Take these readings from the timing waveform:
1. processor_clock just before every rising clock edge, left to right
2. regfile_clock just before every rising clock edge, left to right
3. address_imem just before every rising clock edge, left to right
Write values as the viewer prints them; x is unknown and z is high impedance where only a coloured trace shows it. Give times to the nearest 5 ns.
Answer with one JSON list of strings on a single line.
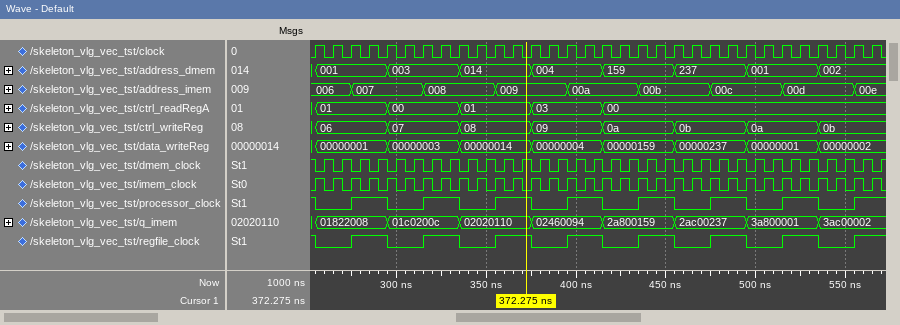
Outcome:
["1 0 0 1 1 0 0 1 1 0 0 1 1 0 0 1 1 0 0 1 1 0 0 1 1 0 0 1 1 0 0 1", "1 0 0 1 1 0 0 1 1 0 0 1 1 0 0 1 1 0 0 1 1 0 0 1 1 0 0 1 1 0 0 1", "006, 006, 006, 007, 007, 007, 007, 008, 008, 008, 008, 009, 009, 009, 009, 00a, 00a, 00a, 00a, 00b, 00b, 00b, 00b, 00c, 00c, 00c, 00c, 00d, 00d, 00d, 00d, 00e"]
